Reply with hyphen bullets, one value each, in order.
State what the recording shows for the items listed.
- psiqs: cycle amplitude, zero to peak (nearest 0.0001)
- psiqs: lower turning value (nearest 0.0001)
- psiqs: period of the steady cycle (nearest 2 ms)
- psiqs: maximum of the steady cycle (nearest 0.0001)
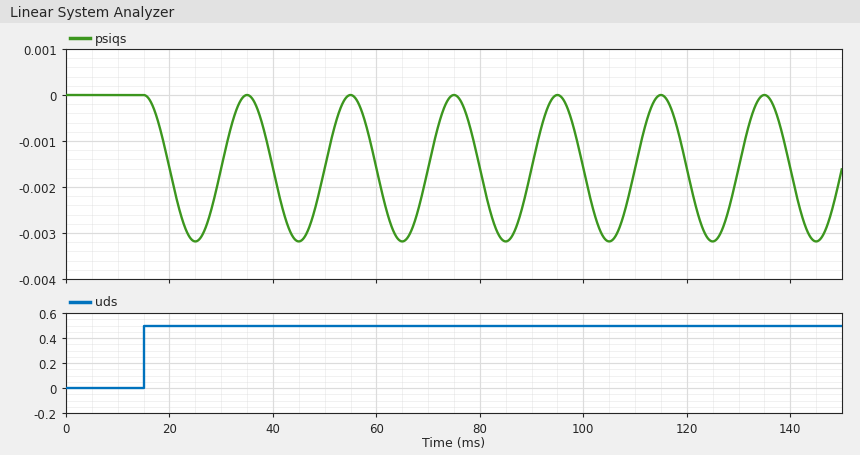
- 0.0016
- -0.0032
- 20 ms
- 0.0000
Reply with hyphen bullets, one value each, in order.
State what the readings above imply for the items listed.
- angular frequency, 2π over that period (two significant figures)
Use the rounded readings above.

- 0.31 rad/ms
